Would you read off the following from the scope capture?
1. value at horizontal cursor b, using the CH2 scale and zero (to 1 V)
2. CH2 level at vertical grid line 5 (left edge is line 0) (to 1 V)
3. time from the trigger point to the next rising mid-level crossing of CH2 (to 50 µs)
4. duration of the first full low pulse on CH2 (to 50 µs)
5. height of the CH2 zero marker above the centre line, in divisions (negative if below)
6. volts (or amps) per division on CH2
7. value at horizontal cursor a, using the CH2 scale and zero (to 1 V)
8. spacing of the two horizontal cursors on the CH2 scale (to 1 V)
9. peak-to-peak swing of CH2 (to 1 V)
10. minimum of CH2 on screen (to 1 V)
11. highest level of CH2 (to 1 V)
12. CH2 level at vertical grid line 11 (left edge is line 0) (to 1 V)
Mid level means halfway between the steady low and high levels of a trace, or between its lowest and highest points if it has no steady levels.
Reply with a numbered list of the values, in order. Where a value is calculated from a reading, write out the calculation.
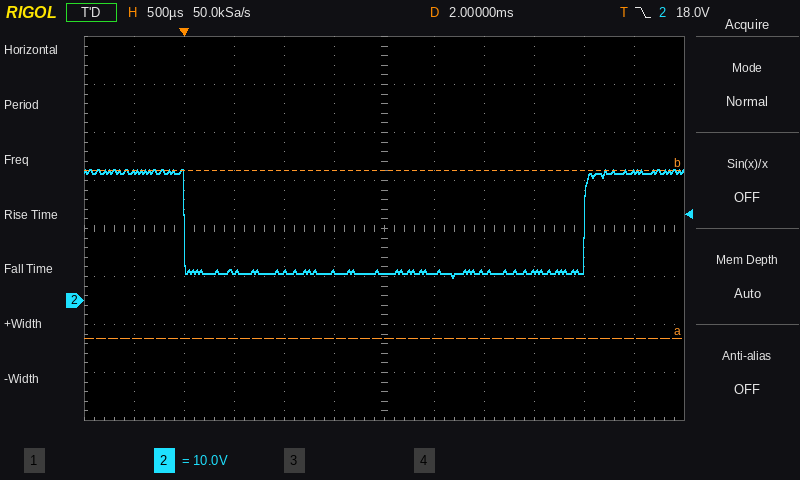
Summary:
1. 27 V
2. 6 V
3. 4.00 ms
4. 4.00 ms
5. -1.5 div
6. 10 V
7. -8 V
8. 35 V
9. 27 V − (5 V) = 22 V
10. 5 V
11. 27 V
12. 27 V
